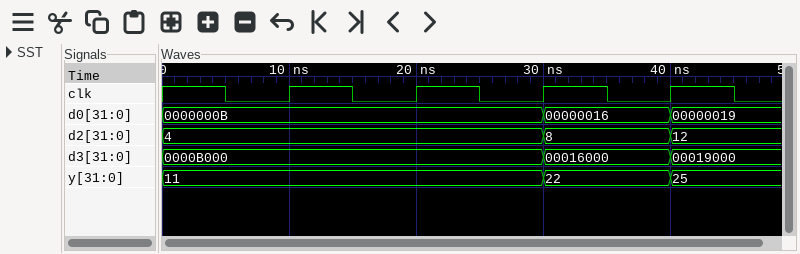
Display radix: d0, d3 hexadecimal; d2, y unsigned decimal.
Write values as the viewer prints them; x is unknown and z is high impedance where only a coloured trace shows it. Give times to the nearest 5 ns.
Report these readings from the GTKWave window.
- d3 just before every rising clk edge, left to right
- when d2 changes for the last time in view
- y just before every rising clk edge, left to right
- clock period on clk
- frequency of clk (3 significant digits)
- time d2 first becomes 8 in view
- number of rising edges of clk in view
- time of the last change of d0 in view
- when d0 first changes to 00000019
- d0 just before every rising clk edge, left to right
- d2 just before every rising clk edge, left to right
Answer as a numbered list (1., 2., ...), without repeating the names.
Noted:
1. 0000B000, 0000B000, 0000B000, 00016000
2. 40 ns
3. 11, 11, 11, 22
4. 10 ns
5. 100 MHz
6. 30 ns
7. 4
8. 40 ns
9. 40 ns
10. 0000000B, 0000000B, 0000000B, 00000016
11. 4, 4, 4, 8
